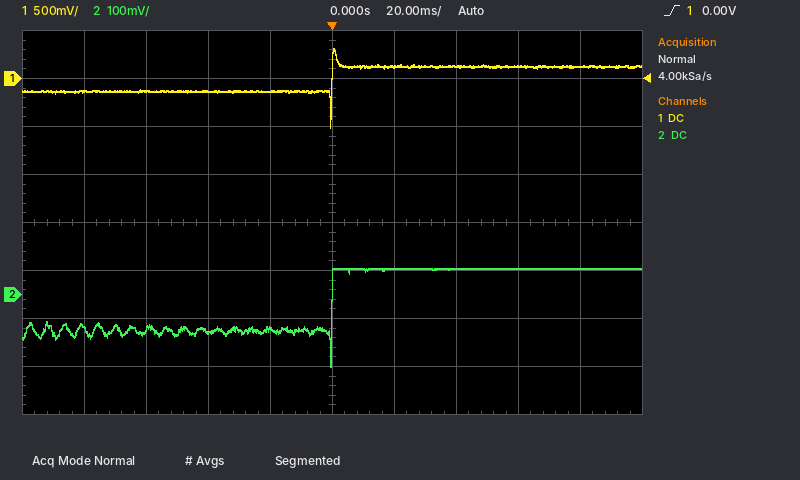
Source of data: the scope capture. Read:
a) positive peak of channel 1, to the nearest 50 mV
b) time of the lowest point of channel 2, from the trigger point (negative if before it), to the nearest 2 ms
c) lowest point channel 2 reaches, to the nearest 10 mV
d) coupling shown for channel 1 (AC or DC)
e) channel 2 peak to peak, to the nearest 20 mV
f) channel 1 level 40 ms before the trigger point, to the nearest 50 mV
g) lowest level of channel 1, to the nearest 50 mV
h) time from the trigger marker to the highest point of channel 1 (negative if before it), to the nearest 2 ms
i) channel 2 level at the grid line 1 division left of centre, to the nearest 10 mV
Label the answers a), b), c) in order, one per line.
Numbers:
a) 300 mV
b) 0 ms
c) -150 mV
d) DC
e) 200 mV
f) -150 mV
g) -500 mV
h) 0 ms
i) -70 mV
